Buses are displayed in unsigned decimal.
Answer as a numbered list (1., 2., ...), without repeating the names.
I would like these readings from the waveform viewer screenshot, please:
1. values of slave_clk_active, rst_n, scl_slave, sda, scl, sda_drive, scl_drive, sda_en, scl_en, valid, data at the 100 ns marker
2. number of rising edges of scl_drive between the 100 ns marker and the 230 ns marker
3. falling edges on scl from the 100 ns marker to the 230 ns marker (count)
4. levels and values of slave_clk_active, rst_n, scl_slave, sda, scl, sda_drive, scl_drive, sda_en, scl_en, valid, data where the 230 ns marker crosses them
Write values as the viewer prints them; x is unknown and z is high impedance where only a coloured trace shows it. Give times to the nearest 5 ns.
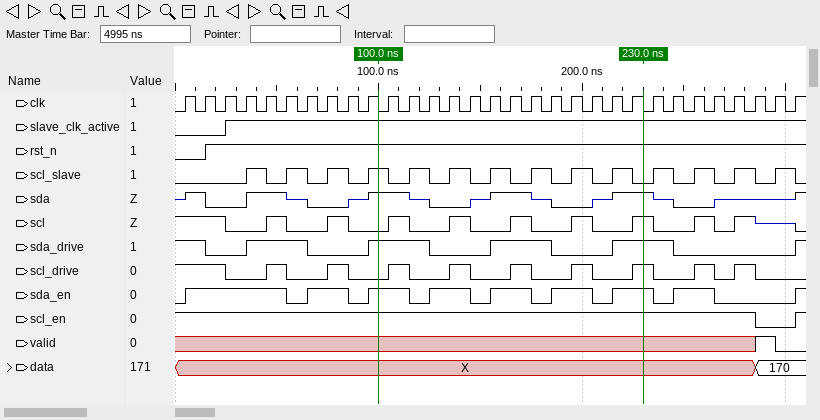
1. slave_clk_active=1, rst_n=1, scl_slave=1, sda=1, scl=0, sda_drive=1, scl_drive=0, sda_en=1, scl_en=1, valid=x, data=X
2. 5
3. 4
4. slave_clk_active=1, rst_n=1, scl_slave=0, sda=1, scl=1, sda_drive=1, scl_drive=1, sda_en=1, scl_en=1, valid=x, data=X
